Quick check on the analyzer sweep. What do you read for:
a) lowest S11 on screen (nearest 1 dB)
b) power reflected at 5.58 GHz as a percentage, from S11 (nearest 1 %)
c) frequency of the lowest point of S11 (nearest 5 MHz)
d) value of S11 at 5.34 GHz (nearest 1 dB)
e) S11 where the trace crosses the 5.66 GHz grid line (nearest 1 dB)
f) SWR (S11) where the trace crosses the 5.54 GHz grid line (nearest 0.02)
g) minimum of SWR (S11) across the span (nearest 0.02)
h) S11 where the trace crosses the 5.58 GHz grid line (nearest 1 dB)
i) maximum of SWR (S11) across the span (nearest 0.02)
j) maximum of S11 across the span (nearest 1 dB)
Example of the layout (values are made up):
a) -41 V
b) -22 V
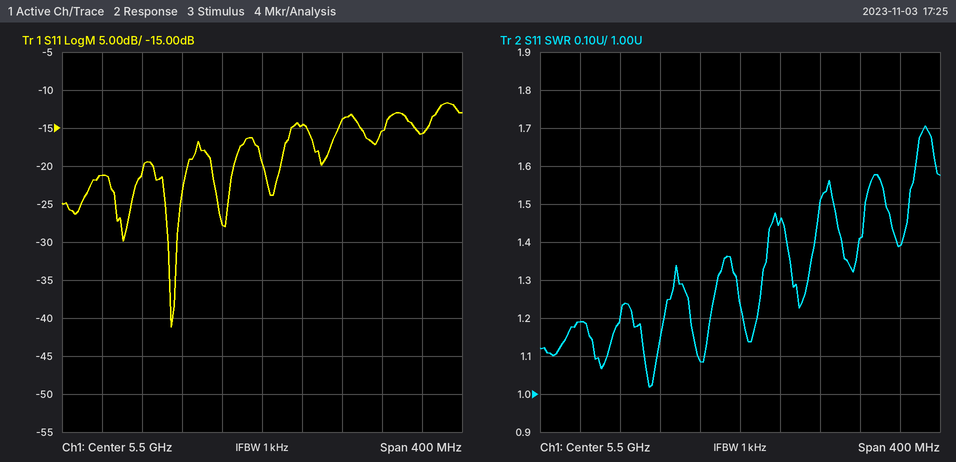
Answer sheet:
a) -41 dB
b) 4 %
c) 5.410 GHz
d) -21 dB
e) -16 dB
f) 1.46
g) 1.02
h) -14 dB
i) 1.70
j) -12 dB
